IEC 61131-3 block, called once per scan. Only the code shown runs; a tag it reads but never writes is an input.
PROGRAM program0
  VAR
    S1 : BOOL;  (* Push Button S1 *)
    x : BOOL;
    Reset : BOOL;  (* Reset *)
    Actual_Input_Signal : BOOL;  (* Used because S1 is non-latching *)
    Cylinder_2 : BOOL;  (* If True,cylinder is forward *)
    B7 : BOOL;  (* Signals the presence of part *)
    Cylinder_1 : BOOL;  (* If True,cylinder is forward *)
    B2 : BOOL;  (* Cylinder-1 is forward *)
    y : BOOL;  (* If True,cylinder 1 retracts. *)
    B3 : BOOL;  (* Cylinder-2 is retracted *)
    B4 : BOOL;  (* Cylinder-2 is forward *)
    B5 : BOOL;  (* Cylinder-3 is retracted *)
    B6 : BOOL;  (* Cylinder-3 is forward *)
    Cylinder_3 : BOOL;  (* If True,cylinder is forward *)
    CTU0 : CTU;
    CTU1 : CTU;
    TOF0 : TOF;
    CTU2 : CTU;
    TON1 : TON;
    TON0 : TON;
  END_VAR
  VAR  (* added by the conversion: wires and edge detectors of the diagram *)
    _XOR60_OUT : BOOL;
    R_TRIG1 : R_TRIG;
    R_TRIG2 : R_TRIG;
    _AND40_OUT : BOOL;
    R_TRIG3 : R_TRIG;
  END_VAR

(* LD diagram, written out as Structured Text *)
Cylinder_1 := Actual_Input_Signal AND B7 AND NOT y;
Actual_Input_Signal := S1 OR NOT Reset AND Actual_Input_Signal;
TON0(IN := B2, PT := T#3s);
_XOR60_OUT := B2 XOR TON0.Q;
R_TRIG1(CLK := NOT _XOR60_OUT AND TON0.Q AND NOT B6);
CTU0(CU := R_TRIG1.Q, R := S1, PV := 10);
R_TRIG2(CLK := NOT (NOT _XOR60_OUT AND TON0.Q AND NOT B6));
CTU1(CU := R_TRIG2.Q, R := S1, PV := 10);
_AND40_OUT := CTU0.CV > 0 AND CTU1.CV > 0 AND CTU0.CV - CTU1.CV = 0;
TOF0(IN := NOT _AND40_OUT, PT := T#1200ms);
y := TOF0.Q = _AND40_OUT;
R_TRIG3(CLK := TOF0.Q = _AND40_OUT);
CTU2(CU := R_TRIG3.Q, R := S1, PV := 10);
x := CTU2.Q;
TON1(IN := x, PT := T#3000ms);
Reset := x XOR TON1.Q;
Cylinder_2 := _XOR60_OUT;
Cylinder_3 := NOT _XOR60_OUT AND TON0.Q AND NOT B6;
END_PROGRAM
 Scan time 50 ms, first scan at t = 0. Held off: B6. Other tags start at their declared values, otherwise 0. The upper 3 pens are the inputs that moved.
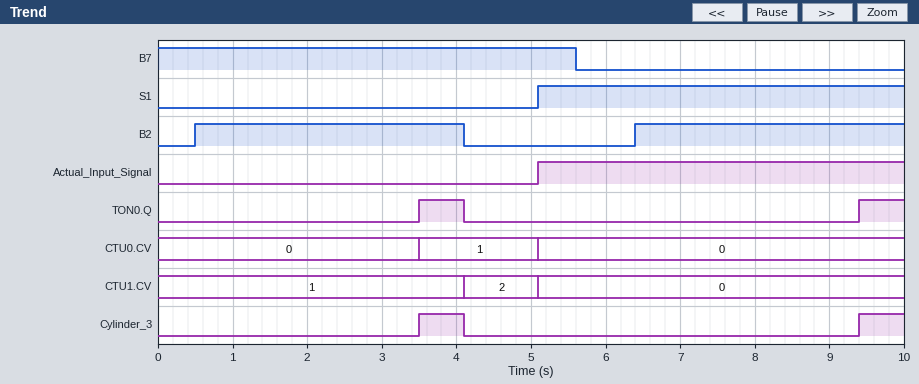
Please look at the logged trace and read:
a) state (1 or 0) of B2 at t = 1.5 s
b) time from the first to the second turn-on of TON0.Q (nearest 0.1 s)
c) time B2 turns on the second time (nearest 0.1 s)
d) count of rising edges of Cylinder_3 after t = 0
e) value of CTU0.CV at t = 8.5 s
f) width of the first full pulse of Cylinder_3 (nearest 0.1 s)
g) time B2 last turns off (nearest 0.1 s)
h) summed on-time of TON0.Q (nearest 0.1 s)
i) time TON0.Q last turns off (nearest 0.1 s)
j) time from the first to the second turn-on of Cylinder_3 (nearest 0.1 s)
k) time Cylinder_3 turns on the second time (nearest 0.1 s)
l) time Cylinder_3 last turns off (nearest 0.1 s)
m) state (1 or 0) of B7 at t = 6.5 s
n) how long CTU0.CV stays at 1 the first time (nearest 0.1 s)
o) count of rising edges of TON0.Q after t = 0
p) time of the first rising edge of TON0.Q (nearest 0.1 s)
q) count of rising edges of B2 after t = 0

1
5.9 s
6.4 s
2
0
0.6 s
4.1 s
1.2 s
4.1 s
5.9 s
9.4 s
4.1 s
0
1.6 s
2
3.5 s
2
